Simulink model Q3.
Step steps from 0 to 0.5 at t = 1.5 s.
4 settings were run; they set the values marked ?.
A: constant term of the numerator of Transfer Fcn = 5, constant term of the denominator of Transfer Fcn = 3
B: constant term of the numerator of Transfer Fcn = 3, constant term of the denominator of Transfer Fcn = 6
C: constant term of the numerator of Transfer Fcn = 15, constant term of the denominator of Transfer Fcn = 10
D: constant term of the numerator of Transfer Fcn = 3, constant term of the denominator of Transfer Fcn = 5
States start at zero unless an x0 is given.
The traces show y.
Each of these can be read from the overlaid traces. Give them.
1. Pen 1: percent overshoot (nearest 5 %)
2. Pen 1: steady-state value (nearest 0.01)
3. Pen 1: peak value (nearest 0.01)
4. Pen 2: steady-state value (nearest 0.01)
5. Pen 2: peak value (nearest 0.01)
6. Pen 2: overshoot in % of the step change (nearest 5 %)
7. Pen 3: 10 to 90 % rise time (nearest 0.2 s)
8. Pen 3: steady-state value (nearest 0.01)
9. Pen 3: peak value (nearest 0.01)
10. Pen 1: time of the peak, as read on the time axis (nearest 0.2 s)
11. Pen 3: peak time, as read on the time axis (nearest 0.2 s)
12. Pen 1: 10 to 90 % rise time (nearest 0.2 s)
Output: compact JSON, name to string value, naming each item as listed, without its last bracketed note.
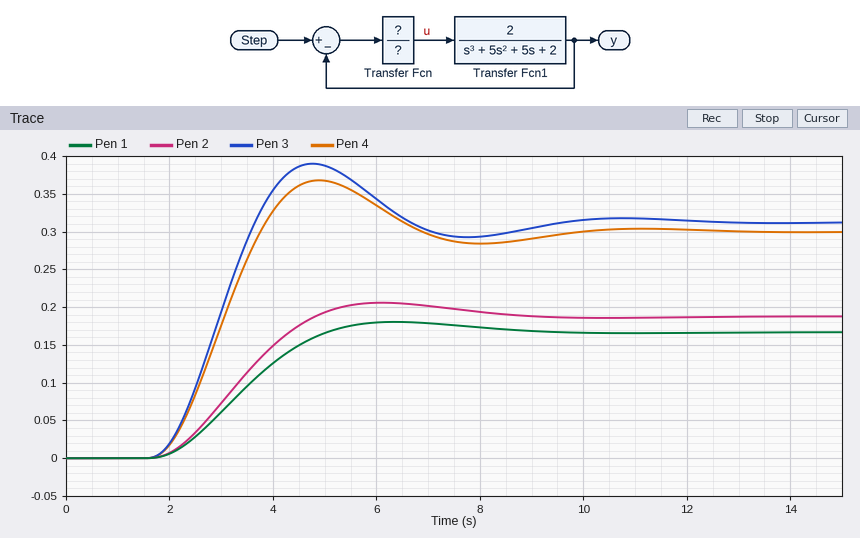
{"Pen 1: percent overshoot": "10 %", "Pen 1: steady-state value": "0.17", "Pen 1: peak value": "0.18", "Pen 2: steady-state value": "0.19", "Pen 2: peak value": "0.21", "Pen 2: overshoot in % of the step change": "10 %", "Pen 3: 10 to 90 % rise time": "1.4 s", "Pen 3: steady-state value": "0.31", "Pen 3: peak value": "0.39", "Pen 1: time of the peak, as read on the time axis": "6.4 s", "Pen 3: peak time, as read on the time axis": "4.8 s", "Pen 1: 10 to 90 % rise time": "2.2 s"}
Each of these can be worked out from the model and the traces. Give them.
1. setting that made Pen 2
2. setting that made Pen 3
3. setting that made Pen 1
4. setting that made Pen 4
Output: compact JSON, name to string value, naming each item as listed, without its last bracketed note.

{"setting that made Pen 2": "D", "setting that made Pen 3": "A", "setting that made Pen 1": "B", "setting that made Pen 4": "C"}
